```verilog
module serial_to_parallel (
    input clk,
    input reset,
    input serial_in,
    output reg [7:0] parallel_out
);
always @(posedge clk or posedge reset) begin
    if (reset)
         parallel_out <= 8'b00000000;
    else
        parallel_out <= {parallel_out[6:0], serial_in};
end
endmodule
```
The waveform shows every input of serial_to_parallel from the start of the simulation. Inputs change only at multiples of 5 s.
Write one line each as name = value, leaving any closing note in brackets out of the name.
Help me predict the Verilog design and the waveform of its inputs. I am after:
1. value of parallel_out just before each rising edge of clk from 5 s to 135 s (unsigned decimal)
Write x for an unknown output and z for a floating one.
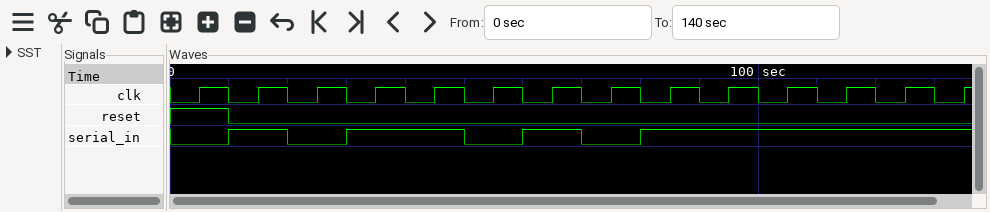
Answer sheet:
value of parallel_out just before each rising edge of clk from 5 s to 135 s = 0, 0, 1, 2, 5, 11, 22, 45, 90, 181, 107, 215, 175, 95
